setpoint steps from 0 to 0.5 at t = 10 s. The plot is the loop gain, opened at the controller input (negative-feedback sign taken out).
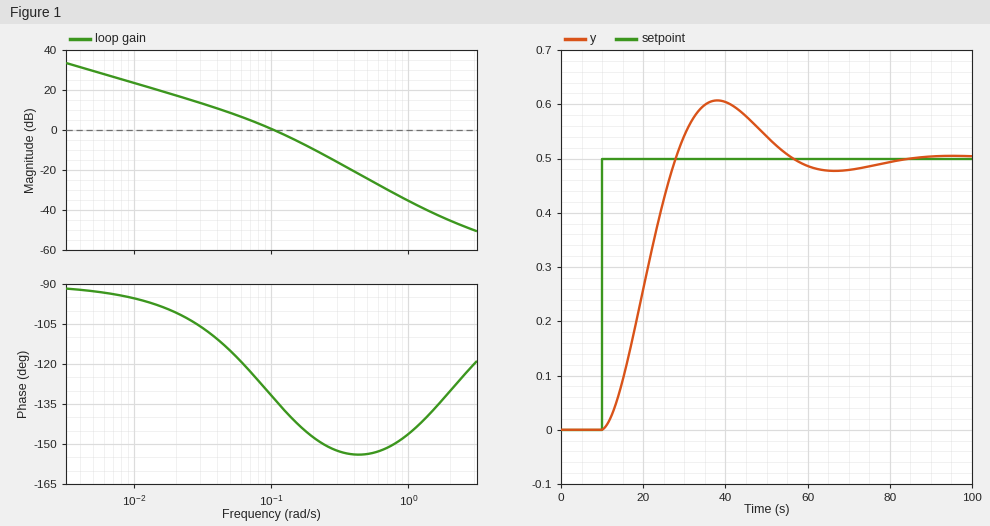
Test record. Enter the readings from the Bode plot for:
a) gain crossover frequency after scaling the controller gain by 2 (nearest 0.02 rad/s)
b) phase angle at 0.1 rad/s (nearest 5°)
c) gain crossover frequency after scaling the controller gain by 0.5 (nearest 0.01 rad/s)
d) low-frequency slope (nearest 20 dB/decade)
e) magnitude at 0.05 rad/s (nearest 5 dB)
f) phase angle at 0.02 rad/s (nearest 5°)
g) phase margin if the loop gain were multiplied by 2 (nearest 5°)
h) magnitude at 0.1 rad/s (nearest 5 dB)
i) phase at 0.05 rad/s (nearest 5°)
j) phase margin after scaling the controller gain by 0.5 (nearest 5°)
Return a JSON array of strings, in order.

["0.16 rad/s", "-130°", "0.06 rad/s", "-20 dB/decade", "10 dB", "-100°", "35°", "0 dB", "-115°", "60°"]
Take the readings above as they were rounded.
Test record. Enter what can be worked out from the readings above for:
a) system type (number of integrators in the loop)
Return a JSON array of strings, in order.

["1"]
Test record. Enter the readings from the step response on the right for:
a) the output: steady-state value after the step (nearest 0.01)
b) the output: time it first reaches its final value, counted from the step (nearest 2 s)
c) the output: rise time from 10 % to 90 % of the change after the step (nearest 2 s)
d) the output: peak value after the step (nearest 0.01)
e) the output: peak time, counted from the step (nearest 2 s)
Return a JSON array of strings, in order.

["0.50", "18 s", "12 s", "0.61", "28 s"]
